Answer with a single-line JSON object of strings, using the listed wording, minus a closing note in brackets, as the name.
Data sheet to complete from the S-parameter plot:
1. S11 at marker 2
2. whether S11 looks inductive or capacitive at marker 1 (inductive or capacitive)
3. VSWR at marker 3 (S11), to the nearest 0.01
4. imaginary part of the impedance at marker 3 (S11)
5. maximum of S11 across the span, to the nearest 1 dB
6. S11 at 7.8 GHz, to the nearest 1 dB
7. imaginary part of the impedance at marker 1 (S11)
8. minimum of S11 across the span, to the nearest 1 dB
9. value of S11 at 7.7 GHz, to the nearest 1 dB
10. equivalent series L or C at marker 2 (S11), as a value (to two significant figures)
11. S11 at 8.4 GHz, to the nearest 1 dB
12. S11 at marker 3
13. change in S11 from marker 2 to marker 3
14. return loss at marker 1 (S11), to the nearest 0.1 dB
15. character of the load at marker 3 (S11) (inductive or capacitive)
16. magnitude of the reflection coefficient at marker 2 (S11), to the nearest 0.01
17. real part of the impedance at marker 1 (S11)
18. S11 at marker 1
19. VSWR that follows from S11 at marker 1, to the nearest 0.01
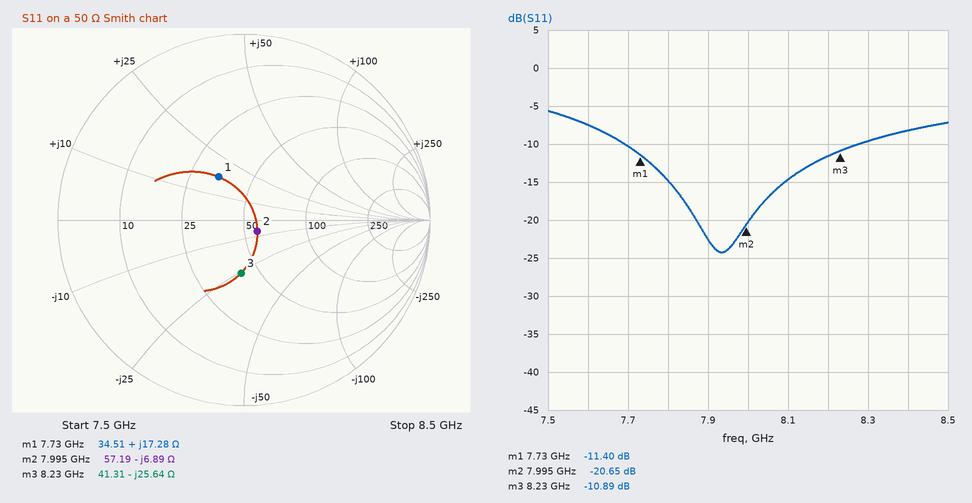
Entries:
{"S11 at marker 2": "-20.65 dB", "whether S11 looks inductive or capacitive at marker 1": "inductive", "VSWR at marker 3 (S11), to the nearest 0.01": "1.80", "imaginary part of the impedance at marker 3": "-25.64 Ω", "maximum of S11 across the span, to the nearest 1 dB": "-6 dB", "S11 at 7.8 GHz, to the nearest 1 dB": "-15 dB", "imaginary part of the impedance at marker 1": "+17.28 Ω", "minimum of S11 across the span, to the nearest 1 dB": "-24 dB", "value of S11 at 7.7 GHz, to the nearest 1 dB": "-10 dB", "equivalent series L or C at marker 2 (S11), as a value": "2.9 pF", "S11 at 8.4 GHz, to the nearest 1 dB": "-8 dB", "S11 at marker 3": "-10.89 dB", "change in S11 from marker 2 to marker 3": "9.76 dB", "return loss at marker 1 (S11), to the nearest 0.1 dB": "11.4 dB", "character of the load at marker 3 (S11)": "capacitive", "magnitude of the reflection coefficient at marker 2 (S11), to the nearest 0.01": "0.09", "real part of the impedance at marker 1": "34.51 Ω", "S11 at marker 1": "-11.40 dB", "VSWR that follows from S11 at marker 1, to the nearest 0.01": "1.74"}
